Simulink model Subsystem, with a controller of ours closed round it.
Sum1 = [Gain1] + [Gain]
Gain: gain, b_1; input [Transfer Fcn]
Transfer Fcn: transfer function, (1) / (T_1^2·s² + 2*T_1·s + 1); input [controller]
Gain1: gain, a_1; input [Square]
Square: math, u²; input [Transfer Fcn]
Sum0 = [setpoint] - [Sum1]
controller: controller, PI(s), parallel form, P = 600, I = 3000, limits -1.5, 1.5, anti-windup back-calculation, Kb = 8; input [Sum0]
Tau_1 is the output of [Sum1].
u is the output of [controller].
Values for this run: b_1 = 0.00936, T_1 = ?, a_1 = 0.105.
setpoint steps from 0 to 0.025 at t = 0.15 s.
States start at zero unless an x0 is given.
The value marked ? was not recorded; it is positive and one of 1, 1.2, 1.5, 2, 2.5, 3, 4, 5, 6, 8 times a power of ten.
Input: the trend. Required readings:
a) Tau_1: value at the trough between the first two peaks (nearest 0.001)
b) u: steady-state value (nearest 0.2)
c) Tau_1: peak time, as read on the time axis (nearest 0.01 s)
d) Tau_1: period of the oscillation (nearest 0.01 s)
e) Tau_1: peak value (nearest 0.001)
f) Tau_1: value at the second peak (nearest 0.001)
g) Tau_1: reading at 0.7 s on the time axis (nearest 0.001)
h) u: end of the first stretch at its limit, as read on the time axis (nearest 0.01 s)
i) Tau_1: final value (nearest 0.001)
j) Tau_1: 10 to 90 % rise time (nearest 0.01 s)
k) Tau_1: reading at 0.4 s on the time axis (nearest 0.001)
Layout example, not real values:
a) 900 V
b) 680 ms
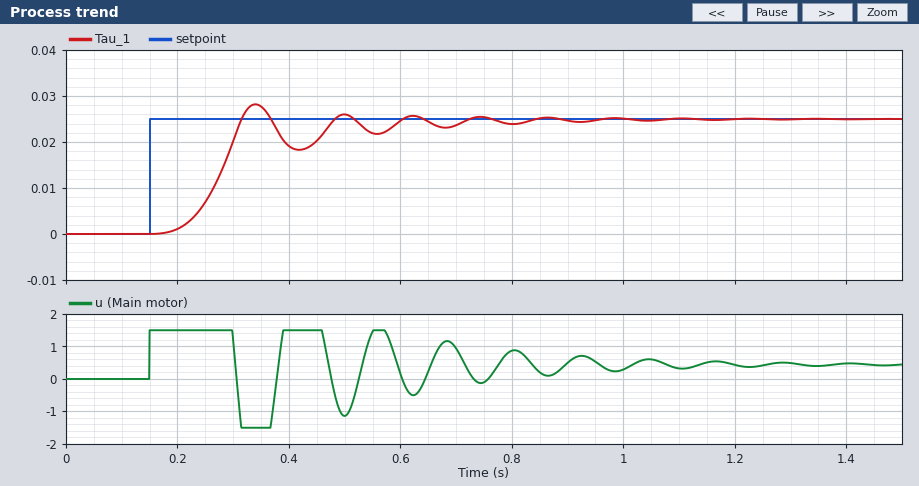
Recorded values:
a) 0.018
b) 0.4
c) 0.34 s
d) 0.16 s
e) 0.028
f) 0.026
g) 0.024
h) 0.30 s
i) 0.025
j) 0.09 s
k) 0.019
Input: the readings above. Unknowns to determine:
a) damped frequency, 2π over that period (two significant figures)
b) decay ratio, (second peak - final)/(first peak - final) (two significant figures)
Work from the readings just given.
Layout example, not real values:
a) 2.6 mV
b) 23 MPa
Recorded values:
a) 39 rad/s
b) 0.33
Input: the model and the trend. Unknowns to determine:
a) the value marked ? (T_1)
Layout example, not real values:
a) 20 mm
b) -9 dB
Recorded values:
a) 0.15
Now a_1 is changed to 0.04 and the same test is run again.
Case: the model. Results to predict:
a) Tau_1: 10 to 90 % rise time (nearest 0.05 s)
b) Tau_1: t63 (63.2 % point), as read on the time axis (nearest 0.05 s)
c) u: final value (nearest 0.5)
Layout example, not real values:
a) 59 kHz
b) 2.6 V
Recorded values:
a) 0.15 s
b) 0.35 s
c) 0.5
